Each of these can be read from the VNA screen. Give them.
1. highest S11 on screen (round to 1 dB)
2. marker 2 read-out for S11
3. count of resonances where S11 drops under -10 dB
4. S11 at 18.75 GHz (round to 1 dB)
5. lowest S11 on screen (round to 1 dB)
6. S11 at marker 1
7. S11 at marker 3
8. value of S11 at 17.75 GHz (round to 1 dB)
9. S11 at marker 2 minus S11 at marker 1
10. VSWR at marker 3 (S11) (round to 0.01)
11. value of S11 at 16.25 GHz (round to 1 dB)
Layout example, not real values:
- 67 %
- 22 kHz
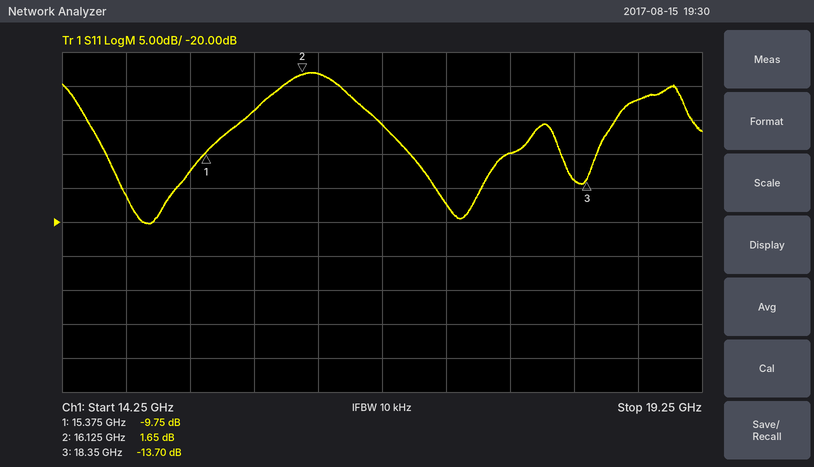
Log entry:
- 2 dB
- 1.65 dB
- 3
- -2 dB
- -20 dB
- -9.75 dB
- -13.70 dB
- -10 dB
- 11.40 dB
- 1.52
- 2 dB
